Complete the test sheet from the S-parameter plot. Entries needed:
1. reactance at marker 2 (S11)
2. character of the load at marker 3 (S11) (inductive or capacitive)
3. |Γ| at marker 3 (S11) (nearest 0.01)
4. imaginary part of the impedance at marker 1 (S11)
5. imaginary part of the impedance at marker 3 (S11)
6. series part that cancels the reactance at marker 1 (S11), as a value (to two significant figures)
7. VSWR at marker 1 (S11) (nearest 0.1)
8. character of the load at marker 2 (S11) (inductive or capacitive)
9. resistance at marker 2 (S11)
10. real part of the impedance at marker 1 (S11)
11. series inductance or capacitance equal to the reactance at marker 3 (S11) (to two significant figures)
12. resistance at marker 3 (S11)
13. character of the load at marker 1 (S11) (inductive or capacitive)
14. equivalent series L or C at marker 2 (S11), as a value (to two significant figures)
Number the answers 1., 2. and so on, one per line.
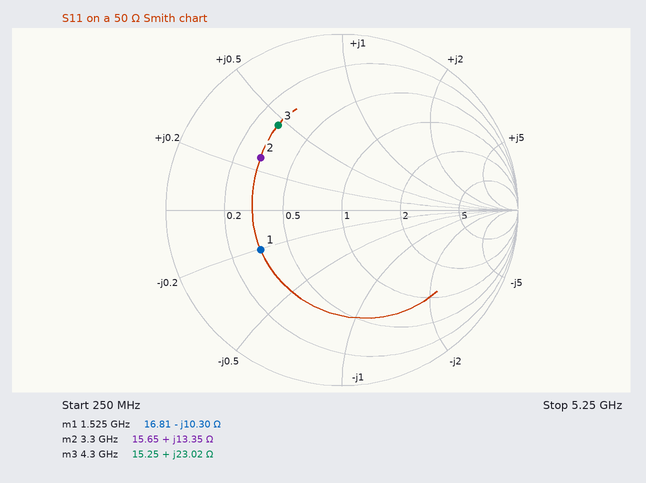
1. +13.35 Ω
2. inductive
3. 0.60
4. -10.30 Ω
5. +23.02 Ω
6. 1.1 nH
7. 3.1
8. inductive
9. 15.65 Ω
10. 16.81 Ω
11. 850 pH
12. 15.25 Ω
13. capacitive
14. 640 pH
